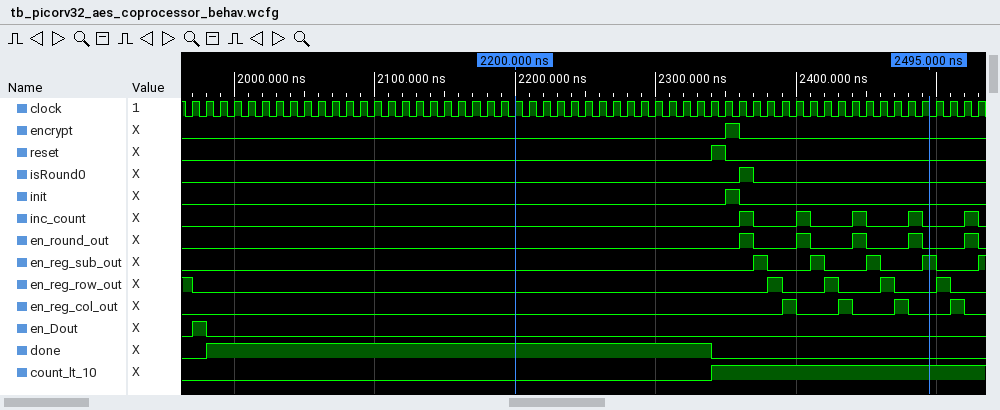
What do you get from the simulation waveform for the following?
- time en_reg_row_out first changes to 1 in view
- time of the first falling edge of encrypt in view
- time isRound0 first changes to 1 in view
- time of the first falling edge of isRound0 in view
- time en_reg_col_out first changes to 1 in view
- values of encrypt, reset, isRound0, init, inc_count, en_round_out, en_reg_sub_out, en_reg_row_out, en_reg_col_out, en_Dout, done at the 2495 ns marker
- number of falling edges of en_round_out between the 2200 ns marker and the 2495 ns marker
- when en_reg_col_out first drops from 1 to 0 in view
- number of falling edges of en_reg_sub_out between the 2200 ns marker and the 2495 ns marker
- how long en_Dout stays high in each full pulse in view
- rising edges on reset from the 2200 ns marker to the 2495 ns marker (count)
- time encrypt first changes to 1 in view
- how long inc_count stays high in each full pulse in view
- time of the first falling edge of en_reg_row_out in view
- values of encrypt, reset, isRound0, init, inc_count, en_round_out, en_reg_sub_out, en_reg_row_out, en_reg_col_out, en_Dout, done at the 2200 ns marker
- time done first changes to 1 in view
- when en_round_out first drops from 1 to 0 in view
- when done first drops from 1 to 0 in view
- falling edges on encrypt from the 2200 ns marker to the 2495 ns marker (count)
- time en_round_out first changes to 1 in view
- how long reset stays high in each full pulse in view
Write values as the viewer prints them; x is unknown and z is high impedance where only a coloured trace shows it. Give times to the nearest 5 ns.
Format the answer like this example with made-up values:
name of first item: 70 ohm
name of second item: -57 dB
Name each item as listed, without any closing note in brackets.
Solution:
time en_reg_row_out first changes to 1 in view: 2380 ns
time of the first falling edge of encrypt in view: 2360 ns
time isRound0 first changes to 1 in view: 2360 ns
time of the first falling edge of isRound0 in view: 2370 ns
time en_reg_col_out first changes to 1 in view: 2390 ns
values of encrypt, reset, isRound0, init, inc_count, en_round_out, en_reg_sub_out, en_reg_row_out, en_reg_col_out, en_Dout, done at the 2495 ns marker: encrypt=0, reset=0, isRound0=0, init=0, inc_count=0, en_round_out=0, en_reg_sub_out=1, en_reg_row_out=0, en_reg_col_out=0, en_Dout=0, done=0
number of falling edges of en_round_out between the 2200 ns marker and the 2495 ns marker: 4
when en_reg_col_out first drops from 1 to 0 in view: 2400 ns
number of falling edges of en_reg_sub_out between the 2200 ns marker and the 2495 ns marker: 3
how long en_Dout stays high in each full pulse in view: 10 ns
rising edges on reset from the 2200 ns marker to the 2495 ns marker: 1
time encrypt first changes to 1 in view: 2350 ns
how long inc_count stays high in each full pulse in view: 10 ns, 10 ns, 10 ns, 10 ns, 10 ns
time of the first falling edge of en_reg_row_out in view: 1970 ns
values of encrypt, reset, isRound0, init, inc_count, en_round_out, en_reg_sub_out, en_reg_row_out, en_reg_col_out, en_Dout, done at the 2200 ns marker: encrypt=0, reset=0, isRound0=0, init=0, inc_count=0, en_round_out=0, en_reg_sub_out=0, en_reg_row_out=0, en_reg_col_out=0, en_Dout=0, done=1
time done first changes to 1 in view: 1980 ns
when en_round_out first drops from 1 to 0 in view: 2370 ns
when done first drops from 1 to 0 in view: 2340 ns
falling edges on encrypt from the 2200 ns marker to the 2495 ns marker: 1
time en_round_out first changes to 1 in view: 2360 ns
how long reset stays high in each full pulse in view: 10 ns
